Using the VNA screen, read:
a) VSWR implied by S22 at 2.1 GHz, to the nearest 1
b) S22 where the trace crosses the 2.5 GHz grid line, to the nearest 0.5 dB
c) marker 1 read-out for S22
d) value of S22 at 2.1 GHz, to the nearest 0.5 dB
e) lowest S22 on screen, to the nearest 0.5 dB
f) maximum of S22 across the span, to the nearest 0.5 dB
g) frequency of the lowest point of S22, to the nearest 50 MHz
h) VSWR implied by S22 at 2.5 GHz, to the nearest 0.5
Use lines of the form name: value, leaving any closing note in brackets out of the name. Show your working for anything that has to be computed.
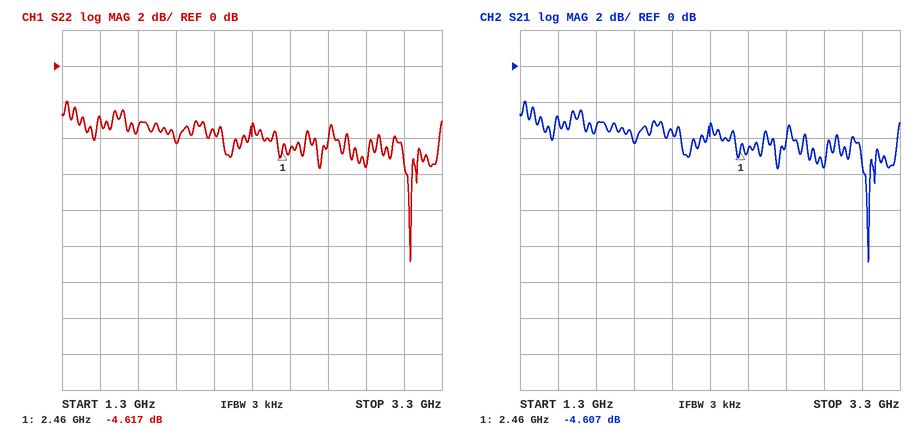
VSWR implied by S22 at 2.1 GHz, to the nearest 1: |Γ| = 10^(-3.5/20) = 0.6683; VSWR = (1 + 0.6683)/(1 − 0.6683) ≈ 5
S22 where the trace crosses the 2.5 GHz grid line, to the nearest 0.5 dB: -4.5 dB
marker 1 read-out for S22: -4.617 dB
value of S22 at 2.1 GHz, to the nearest 0.5 dB: -3.5 dB
lowest S22 on screen, to the nearest 0.5 dB: -11.0 dB
maximum of S22 across the span, to the nearest 0.5 dB: -2.0 dB
frequency of the lowest point of S22, to the nearest 50 MHz: 3.15 GHz
VSWR implied by S22 at 2.5 GHz, to the nearest 0.5: |Γ| = 10^(-4.5/20) = 0.5957; VSWR = (1 + 0.5957)/(1 − 0.5957) ≈ 4.0
